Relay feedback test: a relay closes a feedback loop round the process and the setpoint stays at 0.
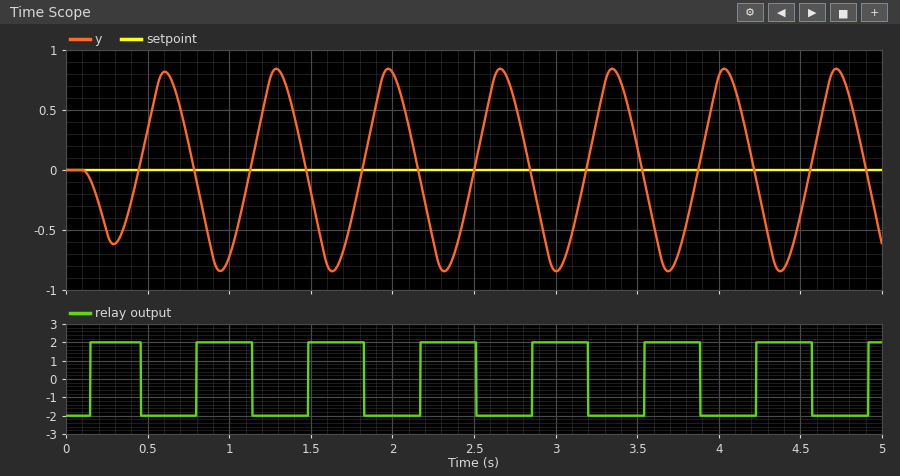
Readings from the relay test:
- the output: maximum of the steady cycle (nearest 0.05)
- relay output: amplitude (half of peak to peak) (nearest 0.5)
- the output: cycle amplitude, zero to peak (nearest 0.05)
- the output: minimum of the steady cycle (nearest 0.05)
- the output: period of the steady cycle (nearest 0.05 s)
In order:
0.85
2.0
0.85
-0.85
0.70 s
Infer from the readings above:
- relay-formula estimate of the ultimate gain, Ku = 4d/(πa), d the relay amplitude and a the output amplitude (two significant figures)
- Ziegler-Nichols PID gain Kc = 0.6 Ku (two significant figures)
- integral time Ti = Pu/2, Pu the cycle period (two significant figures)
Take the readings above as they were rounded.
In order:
3.0
1.8
0.35 s
